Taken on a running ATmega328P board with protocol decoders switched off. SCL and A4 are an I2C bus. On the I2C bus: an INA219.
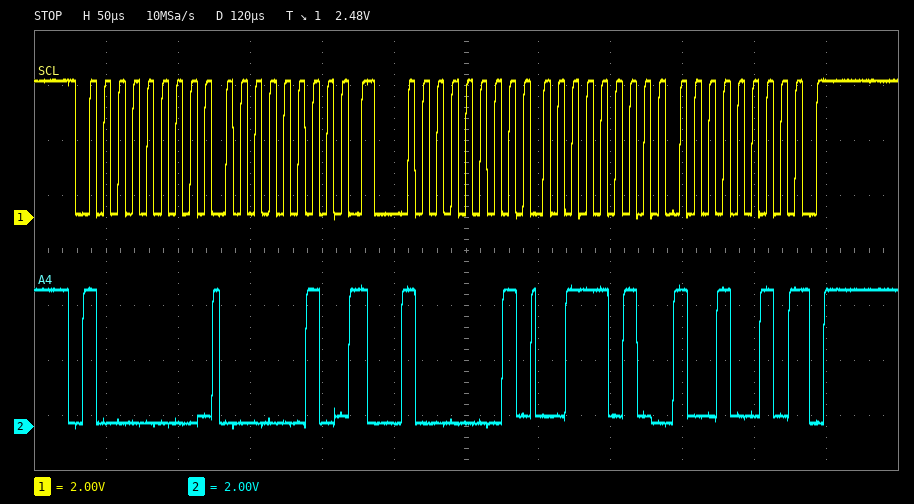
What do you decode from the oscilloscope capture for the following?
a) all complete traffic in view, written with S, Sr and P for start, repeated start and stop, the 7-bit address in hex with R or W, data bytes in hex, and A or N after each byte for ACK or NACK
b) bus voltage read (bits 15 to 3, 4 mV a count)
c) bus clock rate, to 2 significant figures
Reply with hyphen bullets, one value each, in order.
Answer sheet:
- S 40W A 02 A Sr 40R A 3A A 92 N P
- 7.496 V
- 100 kHz
